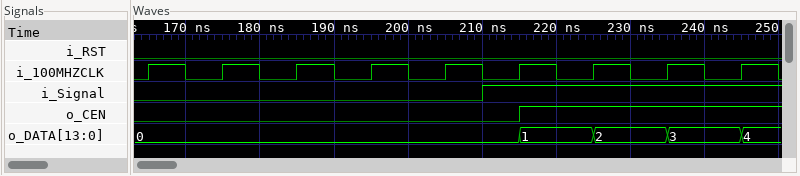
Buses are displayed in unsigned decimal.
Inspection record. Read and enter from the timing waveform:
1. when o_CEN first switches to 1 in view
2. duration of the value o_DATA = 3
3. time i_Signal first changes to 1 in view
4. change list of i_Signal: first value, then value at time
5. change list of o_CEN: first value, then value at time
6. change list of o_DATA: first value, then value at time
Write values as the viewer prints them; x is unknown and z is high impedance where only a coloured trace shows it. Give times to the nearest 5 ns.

215 ns
10 ns
210 ns
0, 1 at 210 ns
0, 1 at 215 ns
0, 1 at 215 ns, 2 at 225 ns, 3 at 235 ns, 4 at 245 ns
